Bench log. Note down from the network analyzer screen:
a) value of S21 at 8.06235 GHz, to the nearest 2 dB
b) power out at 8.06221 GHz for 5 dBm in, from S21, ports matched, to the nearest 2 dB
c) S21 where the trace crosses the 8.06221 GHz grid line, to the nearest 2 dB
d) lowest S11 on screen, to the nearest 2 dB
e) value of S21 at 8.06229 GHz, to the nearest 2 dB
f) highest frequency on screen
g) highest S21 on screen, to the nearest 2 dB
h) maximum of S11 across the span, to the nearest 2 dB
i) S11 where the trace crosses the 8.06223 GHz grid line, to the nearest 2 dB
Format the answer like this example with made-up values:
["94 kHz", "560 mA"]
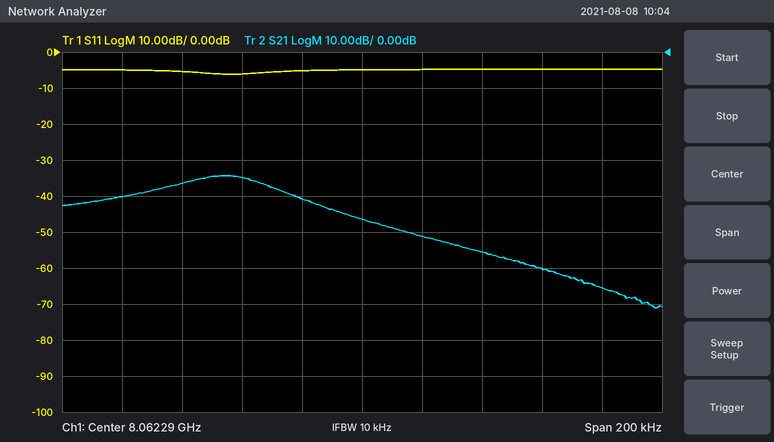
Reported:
["-60 dB", "-36 dBm", "-40 dB", "-6 dB", "-46 dB", "8.06239 GHz", "-34 dB", "-4 dB", "-6 dB"]
